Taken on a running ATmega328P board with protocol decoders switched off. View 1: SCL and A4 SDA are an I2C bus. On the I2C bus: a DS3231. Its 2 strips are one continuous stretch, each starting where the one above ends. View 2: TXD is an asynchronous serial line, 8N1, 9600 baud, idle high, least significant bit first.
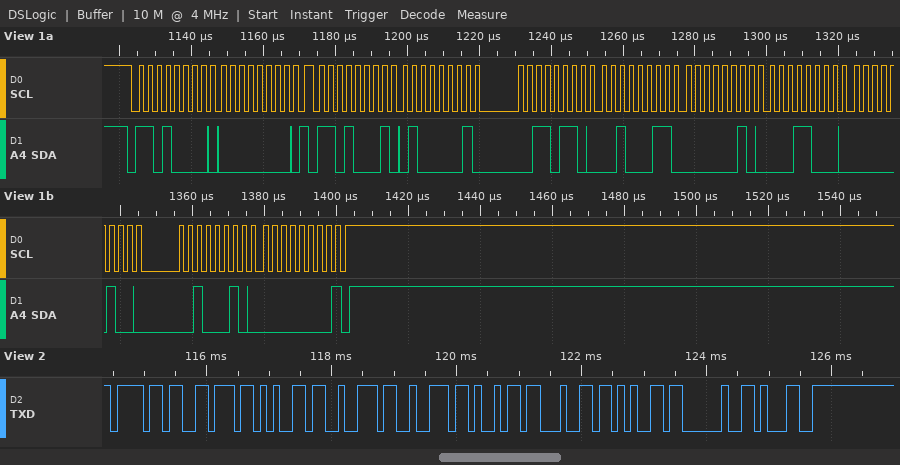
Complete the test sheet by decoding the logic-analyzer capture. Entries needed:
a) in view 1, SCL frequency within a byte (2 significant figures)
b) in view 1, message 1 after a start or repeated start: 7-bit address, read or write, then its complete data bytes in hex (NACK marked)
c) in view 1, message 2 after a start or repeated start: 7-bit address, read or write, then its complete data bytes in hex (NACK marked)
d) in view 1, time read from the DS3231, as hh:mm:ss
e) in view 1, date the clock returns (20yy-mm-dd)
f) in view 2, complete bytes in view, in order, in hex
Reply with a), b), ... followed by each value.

a) 400 kHz
b) 0x68 write: 00
c) 0x68 read: 41 36 23 02 18 04 22 00 NACK
d) 23:36:41
e) 2022-04-18
f) 6F 76 65 72 72 69 64 65 20 31
